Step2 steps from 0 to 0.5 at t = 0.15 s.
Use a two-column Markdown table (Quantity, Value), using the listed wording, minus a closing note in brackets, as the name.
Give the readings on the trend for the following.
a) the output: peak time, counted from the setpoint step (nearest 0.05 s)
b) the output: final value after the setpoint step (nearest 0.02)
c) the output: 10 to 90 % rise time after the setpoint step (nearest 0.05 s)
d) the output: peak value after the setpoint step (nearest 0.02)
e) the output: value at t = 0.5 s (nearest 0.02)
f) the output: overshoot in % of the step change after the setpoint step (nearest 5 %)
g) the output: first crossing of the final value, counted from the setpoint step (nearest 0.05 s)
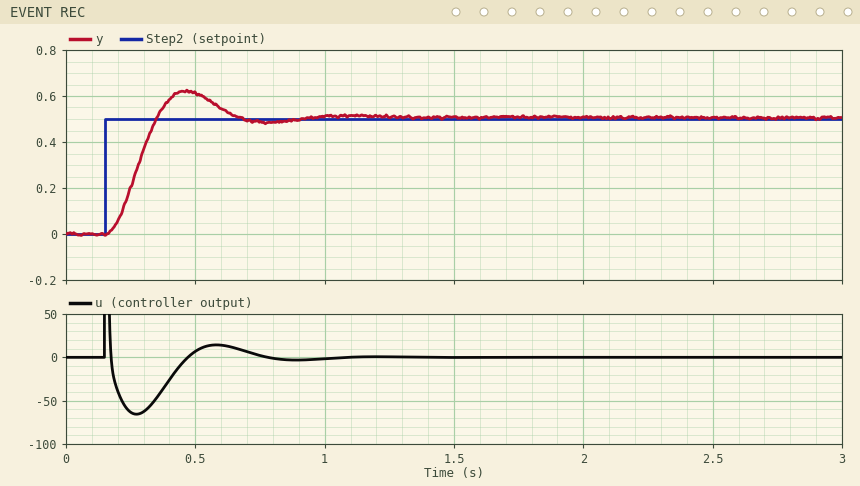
| Quantity | Value |
|---|---|
| the output: peak time, counted from the setpoint step | 0.30 s |
| the output: final value after the setpoint step | 0.50 |
| the output: 10 to 90 % rise time after the setpoint step | 0.15 s |
| the output: peak value after the setpoint step | 0.62 |
| the output: value at t = 0.5 s | 0.62 |
| the output: overshoot in % of the step change after the setpoint step | 25 % |
| the output: first crossing of the final value, counted from the setpoint step | 0.20 s |
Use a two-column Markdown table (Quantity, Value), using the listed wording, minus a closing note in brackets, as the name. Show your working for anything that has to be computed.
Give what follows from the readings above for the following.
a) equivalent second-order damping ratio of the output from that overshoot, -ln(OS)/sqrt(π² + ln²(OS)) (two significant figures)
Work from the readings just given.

| Quantity | Value |
|---|---|
| equivalent second-order damping ratio of the output from that overshoot, -ln(OS)/sqrt(π² + ln²(OS)) | ln(0.25) = -1.386; 1.386 / sqrt(9.870 + 1.922) = 0.40 |
